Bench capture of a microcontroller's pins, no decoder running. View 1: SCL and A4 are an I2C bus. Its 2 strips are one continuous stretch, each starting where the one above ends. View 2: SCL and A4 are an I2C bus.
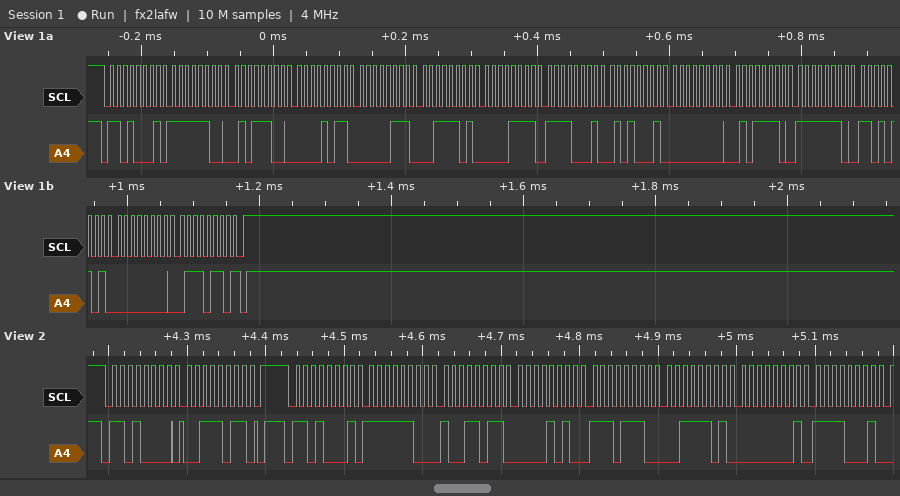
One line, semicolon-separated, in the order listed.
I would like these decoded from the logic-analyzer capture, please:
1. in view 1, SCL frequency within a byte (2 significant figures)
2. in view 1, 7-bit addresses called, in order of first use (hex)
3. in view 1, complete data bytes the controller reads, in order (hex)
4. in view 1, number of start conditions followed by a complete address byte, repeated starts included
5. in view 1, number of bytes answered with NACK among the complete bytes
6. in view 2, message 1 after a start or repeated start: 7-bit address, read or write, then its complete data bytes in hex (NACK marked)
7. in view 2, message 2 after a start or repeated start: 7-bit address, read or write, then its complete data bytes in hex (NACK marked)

100 kHz; 0x68; FC 5C 0B 07 3D 0F F1 51 00 5E FE D5 00 76; 1; 1; 0x68 write: 3B; 0x68 read: FC 9B 0A EE 3D 01 F1
